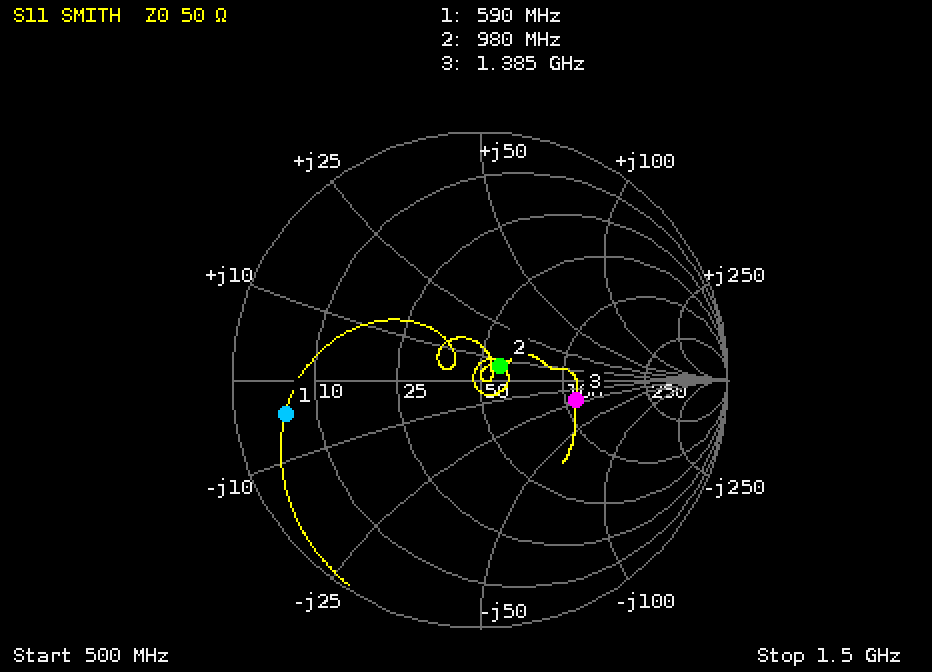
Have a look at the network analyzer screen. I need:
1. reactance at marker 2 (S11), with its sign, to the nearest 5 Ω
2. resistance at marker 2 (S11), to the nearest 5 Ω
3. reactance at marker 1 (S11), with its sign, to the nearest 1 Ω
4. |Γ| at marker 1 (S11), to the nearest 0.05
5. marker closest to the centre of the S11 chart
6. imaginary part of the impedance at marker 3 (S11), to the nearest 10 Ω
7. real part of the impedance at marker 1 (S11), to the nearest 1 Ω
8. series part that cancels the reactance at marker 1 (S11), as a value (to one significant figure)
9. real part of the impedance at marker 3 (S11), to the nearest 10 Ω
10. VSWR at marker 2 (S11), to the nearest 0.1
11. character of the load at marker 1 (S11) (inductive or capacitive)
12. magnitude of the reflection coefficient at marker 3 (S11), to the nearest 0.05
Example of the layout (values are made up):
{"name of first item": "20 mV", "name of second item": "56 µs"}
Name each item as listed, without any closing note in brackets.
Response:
{"reactance at marker 2 (S11), with its sign, to the nearest 5 Ω": "+5 Ω", "resistance at marker 2 (S11), to the nearest 5 Ω": "60 Ω", "reactance at marker 1 (S11), with its sign, to the nearest 1 Ω": "-4 Ω", "|Γ| at marker 1 (S11), to the nearest 0.05": "0.80", "marker closest to the centre of the S11 chart": "marker 2", "imaginary part of the impedance at marker 3 (S11), to the nearest 10 Ω": "-20 Ω", "real part of the impedance at marker 1 (S11), to the nearest 1 Ω": "6 Ω", "series part that cancels the reactance at marker 1 (S11), as a value": "1 nH", "real part of the impedance at marker 3 (S11), to the nearest 10 Ω": "110 Ω", "VSWR at marker 2 (S11), to the nearest 0.1": "1.2", "character of the load at marker 1 (S11)": "capacitive", "magnitude of the reflection coefficient at marker 3 (S11), to the nearest 0.05": "0.40"}
